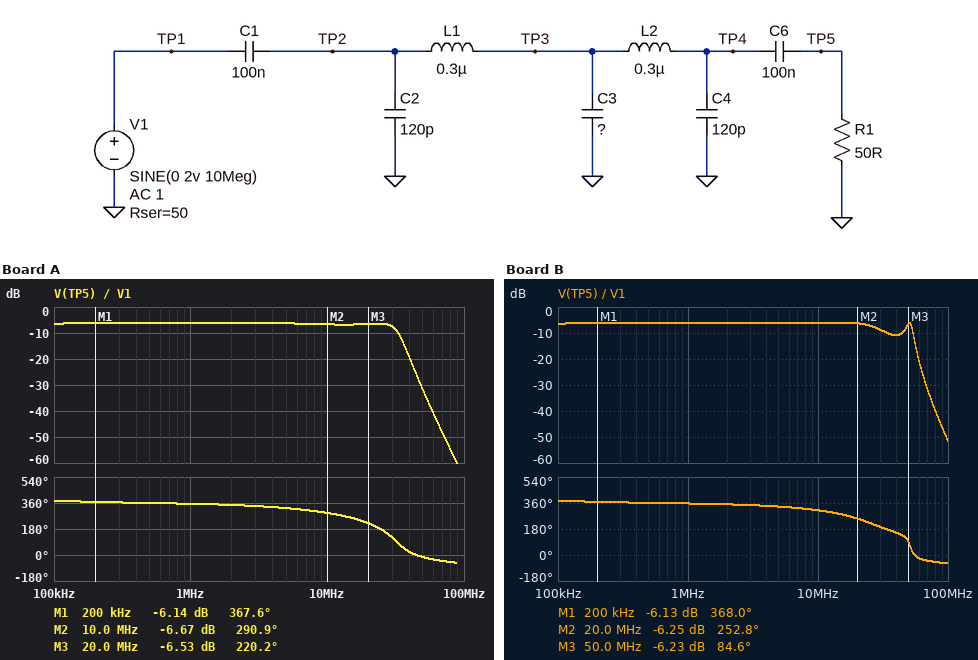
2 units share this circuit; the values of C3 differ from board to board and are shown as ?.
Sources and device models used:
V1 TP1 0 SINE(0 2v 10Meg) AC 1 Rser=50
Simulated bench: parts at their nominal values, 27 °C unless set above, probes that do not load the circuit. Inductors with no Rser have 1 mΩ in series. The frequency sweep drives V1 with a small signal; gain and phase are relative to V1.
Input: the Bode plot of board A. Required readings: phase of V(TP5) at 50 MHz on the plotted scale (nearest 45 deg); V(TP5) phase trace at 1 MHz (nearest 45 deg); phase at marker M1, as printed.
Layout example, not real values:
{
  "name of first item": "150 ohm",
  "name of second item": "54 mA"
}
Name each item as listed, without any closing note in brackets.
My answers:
{
  "phase of V(TP5) at 50 MHz on the plotted scale": "0 deg",
  "V(TP5) phase trace at 1 MHz": "360 deg",
  "phase at marker M1, as printed": "367.6 deg"
}
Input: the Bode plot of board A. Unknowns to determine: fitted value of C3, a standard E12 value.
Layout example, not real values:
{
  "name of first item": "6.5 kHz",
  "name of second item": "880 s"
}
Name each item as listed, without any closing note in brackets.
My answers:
{
  "fitted value of C3, a standard E12 value": "330 pF"
}
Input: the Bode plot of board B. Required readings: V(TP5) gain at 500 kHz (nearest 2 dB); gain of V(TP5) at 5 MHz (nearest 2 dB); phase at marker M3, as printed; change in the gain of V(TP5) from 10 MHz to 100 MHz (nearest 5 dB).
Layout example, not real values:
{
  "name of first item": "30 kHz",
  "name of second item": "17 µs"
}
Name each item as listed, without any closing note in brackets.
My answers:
{
  "V(TP5) gain at 500 kHz": "-6 dB",
  "gain of V(TP5) at 5 MHz": "-6 dB",
  "phase at marker M3, as printed": "84.6 deg",
  "change in the gain of V(TP5) from 10 MHz to 100 MHz": "-45 dB"
}
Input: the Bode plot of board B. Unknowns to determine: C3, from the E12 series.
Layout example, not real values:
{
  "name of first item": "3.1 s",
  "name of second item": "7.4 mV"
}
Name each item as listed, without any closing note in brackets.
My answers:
{
  "C3, from the E12 series": "82 pF"
}
